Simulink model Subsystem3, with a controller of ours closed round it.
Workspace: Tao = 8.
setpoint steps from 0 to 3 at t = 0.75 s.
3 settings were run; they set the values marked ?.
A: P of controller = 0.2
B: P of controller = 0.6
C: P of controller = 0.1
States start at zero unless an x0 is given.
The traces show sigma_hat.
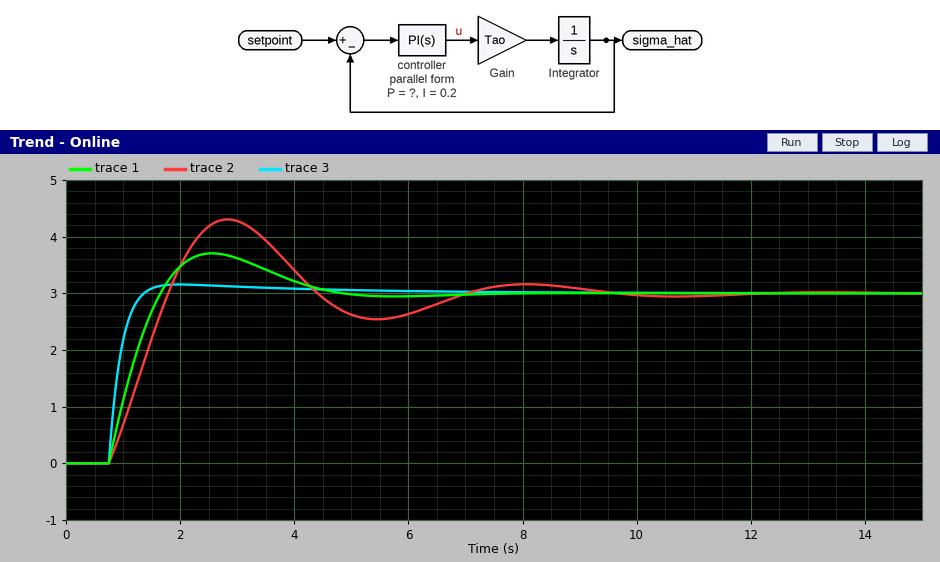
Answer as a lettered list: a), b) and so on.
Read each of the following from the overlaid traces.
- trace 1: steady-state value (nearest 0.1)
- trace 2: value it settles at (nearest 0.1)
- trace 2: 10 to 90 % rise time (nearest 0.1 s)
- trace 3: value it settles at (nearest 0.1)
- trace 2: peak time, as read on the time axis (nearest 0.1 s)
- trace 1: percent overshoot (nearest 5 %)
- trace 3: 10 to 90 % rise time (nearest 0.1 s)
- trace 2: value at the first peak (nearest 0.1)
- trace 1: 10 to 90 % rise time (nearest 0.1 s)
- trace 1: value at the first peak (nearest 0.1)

a) 3.0
b) 3.0
c) 0.8 s
d) 3.0
e) 2.8 s
f) 25 %
g) 0.4 s
h) 4.3
i) 0.7 s
j) 3.7
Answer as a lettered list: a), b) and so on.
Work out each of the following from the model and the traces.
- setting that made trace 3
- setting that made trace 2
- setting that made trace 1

a) B
b) C
c) A
